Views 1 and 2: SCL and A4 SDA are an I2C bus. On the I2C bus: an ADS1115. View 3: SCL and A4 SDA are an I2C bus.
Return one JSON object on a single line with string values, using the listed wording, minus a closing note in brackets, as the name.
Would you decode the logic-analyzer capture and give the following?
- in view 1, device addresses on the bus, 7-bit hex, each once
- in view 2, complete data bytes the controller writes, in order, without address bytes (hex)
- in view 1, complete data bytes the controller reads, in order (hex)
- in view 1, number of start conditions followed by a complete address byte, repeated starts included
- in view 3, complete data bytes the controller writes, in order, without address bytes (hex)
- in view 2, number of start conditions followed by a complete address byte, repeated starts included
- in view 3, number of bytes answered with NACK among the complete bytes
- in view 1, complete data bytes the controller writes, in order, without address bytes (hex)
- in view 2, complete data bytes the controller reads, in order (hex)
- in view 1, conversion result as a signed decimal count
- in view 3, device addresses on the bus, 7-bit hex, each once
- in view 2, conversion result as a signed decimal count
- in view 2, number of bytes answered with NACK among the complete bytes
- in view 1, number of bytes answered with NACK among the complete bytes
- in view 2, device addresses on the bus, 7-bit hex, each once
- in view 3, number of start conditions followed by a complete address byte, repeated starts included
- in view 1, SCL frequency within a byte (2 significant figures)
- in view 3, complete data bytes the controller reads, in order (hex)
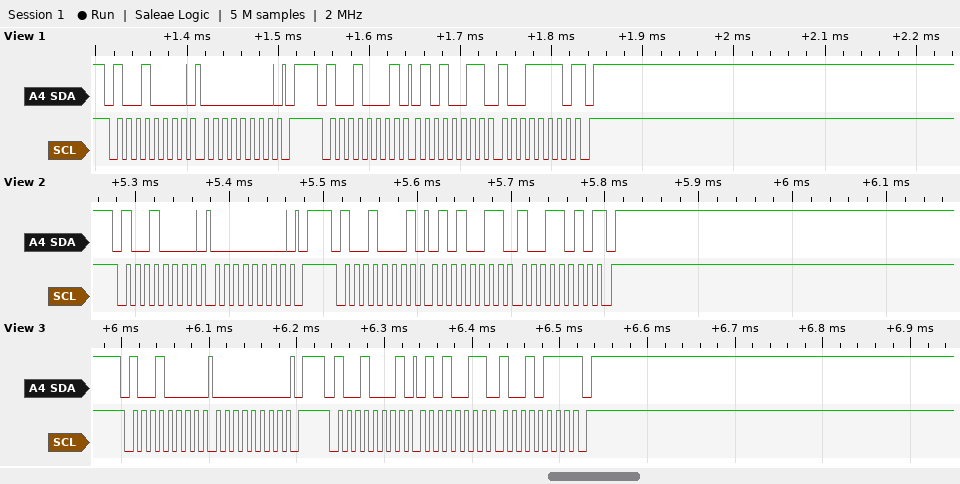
{"in view 1, device addresses on the bus, 7-bit hex, each once": "0x48", "in view 2, complete data bytes the controller writes, in order, without address bytes": "00", "in view 1, complete data bytes the controller reads, in order": "53 9E", "in view 1, number of start conditions followed by a complete address byte, repeated starts included": "2", "in view 3, complete data bytes the controller writes, in order, without address bytes": "00", "in view 2, number of start conditions followed by a complete address byte, repeated starts included": "2", "in view 3, number of bytes answered with NACK among the complete bytes": "1", "in view 1, complete data bytes the controller writes, in order, without address bytes": "00", "in view 2, complete data bytes the controller reads, in order": "53 9A", "in view 1, conversion result as a signed decimal count": "21406", "in view 3, device addresses on the bus, 7-bit hex, each once": "0x48", "in view 2, conversion result as a signed decimal count": "21402", "in view 2, number of bytes answered with NACK among the complete bytes": "1", "in view 1, number of bytes answered with NACK among the complete bytes": "1", "in view 2, device addresses on the bus, 7-bit hex, each once": "0x48", "in view 3, number of start conditions followed by a complete address byte, repeated starts included": "2", "in view 1, SCL frequency within a byte": "100 kHz", "in view 3, complete data bytes the controller reads, in order": "53 97"}
